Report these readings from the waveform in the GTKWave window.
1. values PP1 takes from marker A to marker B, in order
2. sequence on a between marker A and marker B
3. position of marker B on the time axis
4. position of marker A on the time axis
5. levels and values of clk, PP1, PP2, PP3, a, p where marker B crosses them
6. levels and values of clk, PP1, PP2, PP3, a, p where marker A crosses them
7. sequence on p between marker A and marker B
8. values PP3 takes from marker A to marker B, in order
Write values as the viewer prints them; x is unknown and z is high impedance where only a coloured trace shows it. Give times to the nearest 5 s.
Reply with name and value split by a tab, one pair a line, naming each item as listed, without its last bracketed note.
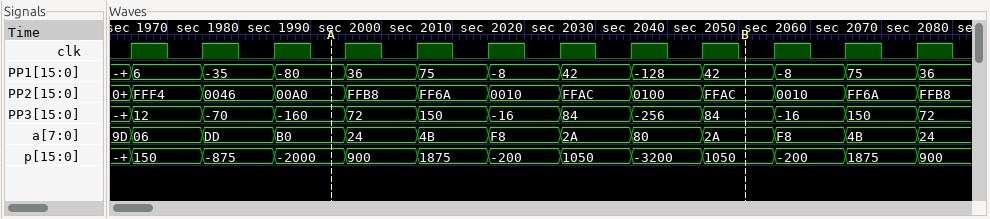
values PP1 takes from marker A to marker B, in order	-80, 36, 75, -8, 42, -128, 42
sequence on a between marker A and marker B	B0, 24, 4B, F8, 2A, 80, 2A
position of marker B on the time axis	2050 s
position of marker A on the time axis	1995 s
levels and values of clk, PP1, PP2, PP3, a, p where marker B crosses them	clk=0, PP1=42, PP2=FFAC, PP3=84, a=2A, p=1050
levels and values of clk, PP1, PP2, PP3, a, p where marker A crosses them	clk=0, PP1=-80, PP2=00A0, PP3=-160, a=B0, p=-2000
sequence on p between marker A and marker B	-2000, 900, 1875, -200, 1050, -3200, 1050
values PP3 takes from marker A to marker B, in order	-160, 72, 150, -16, 84, -256, 84
